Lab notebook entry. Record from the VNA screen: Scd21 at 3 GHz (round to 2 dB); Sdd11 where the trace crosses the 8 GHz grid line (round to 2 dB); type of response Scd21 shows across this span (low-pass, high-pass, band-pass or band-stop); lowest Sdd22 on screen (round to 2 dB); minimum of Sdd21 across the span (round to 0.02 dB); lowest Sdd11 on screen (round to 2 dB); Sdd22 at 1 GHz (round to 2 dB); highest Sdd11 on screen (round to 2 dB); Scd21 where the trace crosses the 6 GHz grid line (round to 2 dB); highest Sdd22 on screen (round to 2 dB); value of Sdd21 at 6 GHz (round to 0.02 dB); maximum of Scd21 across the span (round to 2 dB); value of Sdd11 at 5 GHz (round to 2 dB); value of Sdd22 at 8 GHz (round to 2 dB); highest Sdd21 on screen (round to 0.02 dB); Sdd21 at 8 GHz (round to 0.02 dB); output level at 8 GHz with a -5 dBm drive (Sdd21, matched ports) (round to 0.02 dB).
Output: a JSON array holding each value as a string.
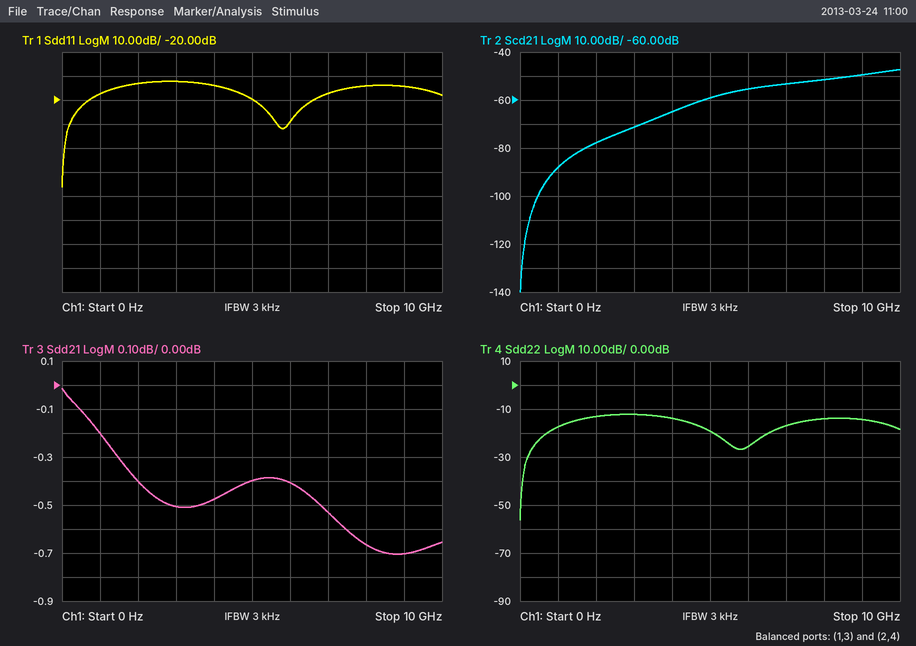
["-72 dB", "-14 dB", "high-pass", "-56 dB", "-0.70 dB", "-56 dB", "-18 dB", "-12 dB", "-56 dB", "-12 dB", "-0.40 dB", "-48 dB", "-20 dB", "-14 dB", "-0.02 dB", "-0.66 dB", "-5.66 dBm"]
